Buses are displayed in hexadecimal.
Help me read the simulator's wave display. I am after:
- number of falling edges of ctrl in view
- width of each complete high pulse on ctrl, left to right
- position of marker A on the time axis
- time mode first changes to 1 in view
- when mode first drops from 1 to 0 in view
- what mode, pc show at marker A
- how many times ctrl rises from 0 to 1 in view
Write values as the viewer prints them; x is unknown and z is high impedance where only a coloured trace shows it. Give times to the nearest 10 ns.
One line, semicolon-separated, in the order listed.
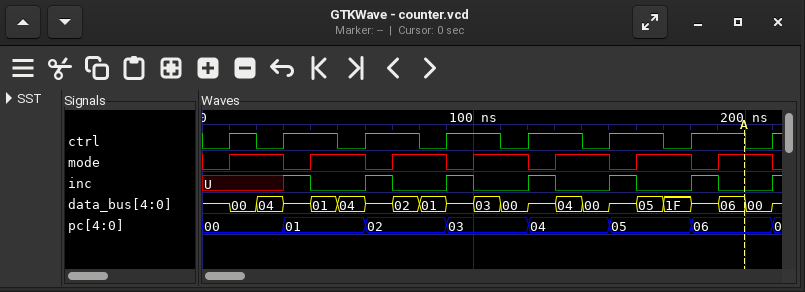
7; 10 ns, 20 ns, 20 ns, 20 ns, 20 ns, 20 ns, 20 ns; 200 ns; 10 ns; 30 ns; mode=1, pc=06; 8
